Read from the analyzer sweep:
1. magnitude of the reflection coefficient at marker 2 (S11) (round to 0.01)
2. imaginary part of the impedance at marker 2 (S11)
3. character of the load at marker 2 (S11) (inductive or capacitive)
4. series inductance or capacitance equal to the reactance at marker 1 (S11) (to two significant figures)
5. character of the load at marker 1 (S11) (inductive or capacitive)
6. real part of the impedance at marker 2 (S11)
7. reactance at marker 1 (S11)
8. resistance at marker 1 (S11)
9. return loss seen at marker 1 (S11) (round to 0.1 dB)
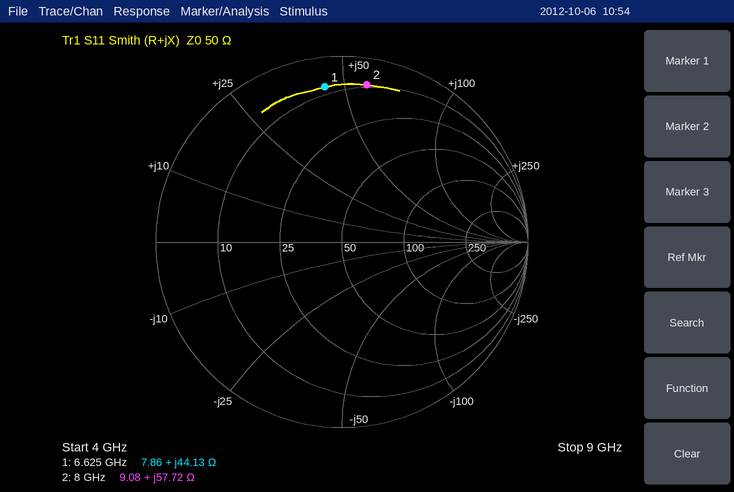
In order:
0.86
+57.72 Ω
inductive
1.1 nH
inductive
9.08 Ω
+44.13 Ω
7.86 Ω
1.5 dB
